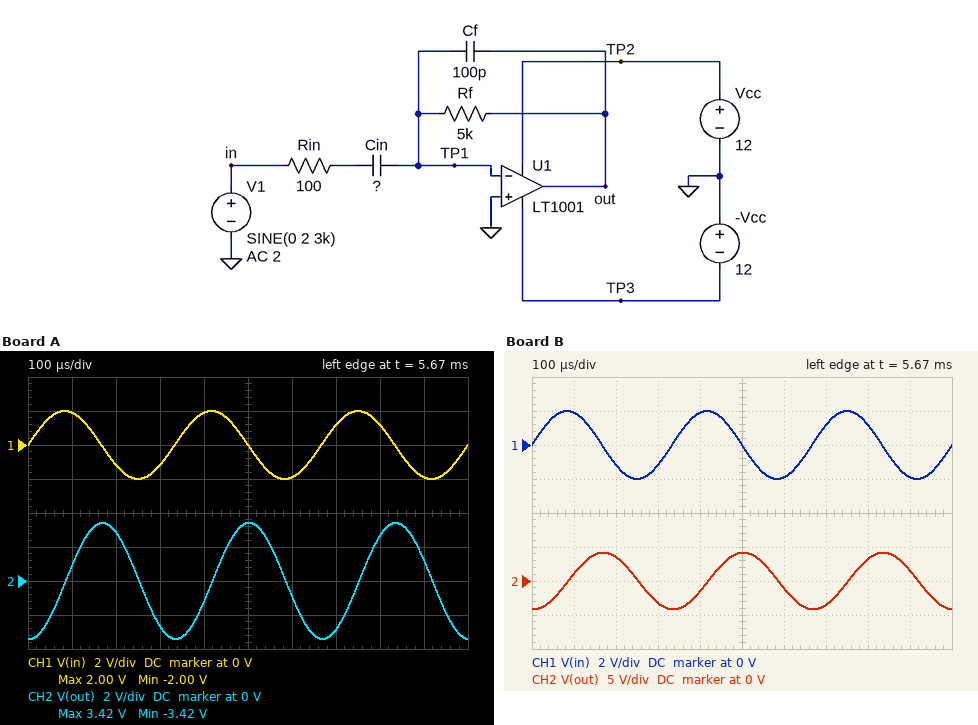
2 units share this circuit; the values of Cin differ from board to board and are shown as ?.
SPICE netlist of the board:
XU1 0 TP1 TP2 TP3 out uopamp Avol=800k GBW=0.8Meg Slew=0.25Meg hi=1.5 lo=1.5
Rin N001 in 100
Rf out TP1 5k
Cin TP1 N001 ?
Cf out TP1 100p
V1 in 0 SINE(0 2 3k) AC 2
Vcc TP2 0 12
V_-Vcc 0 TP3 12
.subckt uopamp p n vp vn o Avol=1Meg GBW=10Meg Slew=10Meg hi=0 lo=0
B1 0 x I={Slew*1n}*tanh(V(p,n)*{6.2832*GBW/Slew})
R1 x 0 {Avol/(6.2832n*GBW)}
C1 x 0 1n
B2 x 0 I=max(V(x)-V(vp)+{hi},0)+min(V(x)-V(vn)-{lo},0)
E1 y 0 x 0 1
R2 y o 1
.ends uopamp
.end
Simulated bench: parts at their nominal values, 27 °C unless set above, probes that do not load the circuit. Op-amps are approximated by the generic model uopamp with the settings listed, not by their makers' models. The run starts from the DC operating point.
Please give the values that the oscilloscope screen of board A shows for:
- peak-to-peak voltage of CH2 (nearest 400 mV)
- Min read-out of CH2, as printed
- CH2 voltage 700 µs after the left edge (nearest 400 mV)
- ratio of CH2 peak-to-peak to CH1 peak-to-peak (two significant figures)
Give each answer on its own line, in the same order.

6.8 V
-3.42 V
-2.8 V
1.7
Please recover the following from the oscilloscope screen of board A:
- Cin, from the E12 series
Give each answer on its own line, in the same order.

18 nF
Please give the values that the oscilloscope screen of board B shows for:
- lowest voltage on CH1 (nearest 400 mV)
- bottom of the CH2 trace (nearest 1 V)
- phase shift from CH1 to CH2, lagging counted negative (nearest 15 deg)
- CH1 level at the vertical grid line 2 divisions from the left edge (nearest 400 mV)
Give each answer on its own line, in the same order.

-2.0 V
-4 V
-90 deg
-1.2 V
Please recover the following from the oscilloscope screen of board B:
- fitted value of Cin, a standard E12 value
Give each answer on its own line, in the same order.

22 nF
